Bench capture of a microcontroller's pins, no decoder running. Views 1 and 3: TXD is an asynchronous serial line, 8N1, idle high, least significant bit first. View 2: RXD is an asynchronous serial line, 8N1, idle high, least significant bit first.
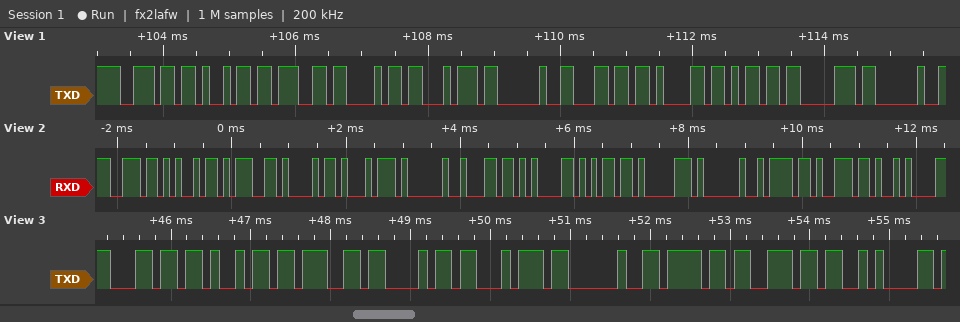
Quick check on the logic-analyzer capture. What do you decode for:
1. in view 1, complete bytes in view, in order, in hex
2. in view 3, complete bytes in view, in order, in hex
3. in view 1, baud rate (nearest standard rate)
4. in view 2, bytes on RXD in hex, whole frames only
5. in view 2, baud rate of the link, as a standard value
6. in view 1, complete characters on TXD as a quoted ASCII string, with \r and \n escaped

0x6E 0x69 0x67 0x68 0x74 0x20 0x6C 0x61 0x6D 0x70 0x20
6C 69 67 68 74 20 6F 6E 0A
9600 baud
6E 69 67 68 74 20 6C 61 6D 70 20 6F 6E 0A
9600 baud
"night lamp "
